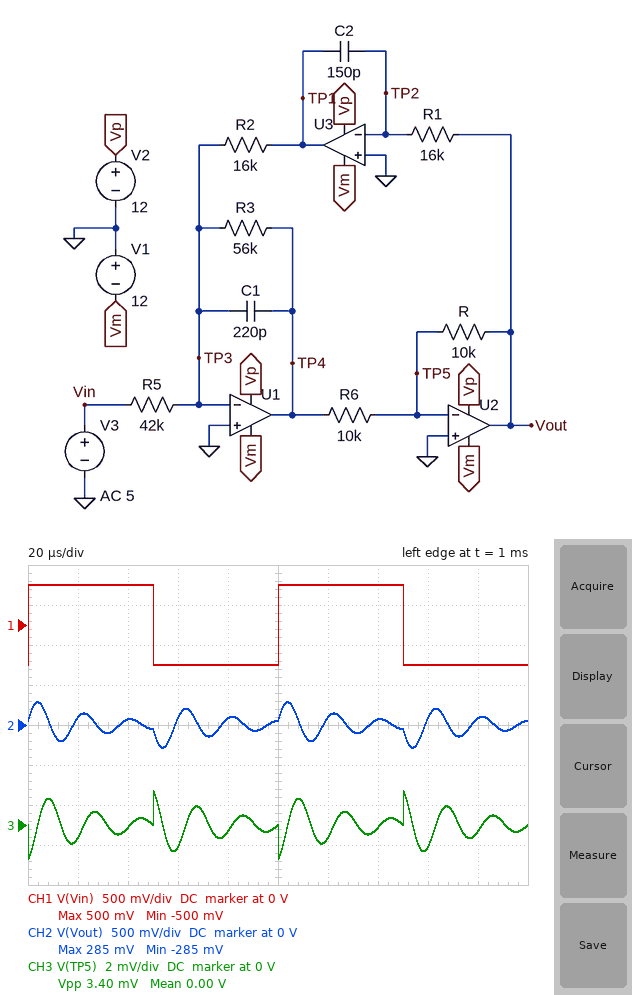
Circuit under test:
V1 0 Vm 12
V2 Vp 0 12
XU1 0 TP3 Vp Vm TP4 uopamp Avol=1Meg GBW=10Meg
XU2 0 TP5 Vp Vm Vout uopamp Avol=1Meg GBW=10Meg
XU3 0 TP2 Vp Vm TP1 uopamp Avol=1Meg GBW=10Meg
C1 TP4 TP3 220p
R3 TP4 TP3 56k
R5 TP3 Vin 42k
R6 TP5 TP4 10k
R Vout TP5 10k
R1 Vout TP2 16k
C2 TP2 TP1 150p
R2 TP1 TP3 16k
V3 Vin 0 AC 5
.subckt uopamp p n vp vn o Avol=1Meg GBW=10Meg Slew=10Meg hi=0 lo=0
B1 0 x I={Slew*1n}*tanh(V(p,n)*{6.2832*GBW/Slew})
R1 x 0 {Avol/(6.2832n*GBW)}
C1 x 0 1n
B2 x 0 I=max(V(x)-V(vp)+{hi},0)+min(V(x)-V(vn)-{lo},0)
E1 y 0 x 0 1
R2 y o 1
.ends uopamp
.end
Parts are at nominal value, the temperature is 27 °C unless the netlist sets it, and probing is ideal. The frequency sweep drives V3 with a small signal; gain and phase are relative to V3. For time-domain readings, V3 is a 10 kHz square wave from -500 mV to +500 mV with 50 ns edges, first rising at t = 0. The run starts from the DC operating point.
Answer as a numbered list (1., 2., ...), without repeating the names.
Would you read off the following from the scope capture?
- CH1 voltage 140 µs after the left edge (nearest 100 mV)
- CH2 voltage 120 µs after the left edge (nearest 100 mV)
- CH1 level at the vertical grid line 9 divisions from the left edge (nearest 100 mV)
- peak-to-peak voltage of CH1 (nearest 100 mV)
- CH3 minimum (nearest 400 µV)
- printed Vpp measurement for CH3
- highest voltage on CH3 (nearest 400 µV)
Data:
1. 500 mV
2. 100 mV
3. -500 mV
4. 1.0 V
5. -1.6 mV
6. 3.40 mV
7. 1.6 mV
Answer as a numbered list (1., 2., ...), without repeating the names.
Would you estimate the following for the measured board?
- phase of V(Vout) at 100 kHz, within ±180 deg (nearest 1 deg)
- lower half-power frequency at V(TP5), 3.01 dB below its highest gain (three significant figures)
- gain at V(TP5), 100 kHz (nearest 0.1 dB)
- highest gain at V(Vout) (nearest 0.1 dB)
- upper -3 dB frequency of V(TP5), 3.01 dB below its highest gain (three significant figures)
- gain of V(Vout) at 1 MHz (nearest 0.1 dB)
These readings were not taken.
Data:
1. -82 deg
2. 49.9 kHz
3. -52.4 dB
4. 3.3 dB
5. 62.2 kHz
6. -35.5 dB
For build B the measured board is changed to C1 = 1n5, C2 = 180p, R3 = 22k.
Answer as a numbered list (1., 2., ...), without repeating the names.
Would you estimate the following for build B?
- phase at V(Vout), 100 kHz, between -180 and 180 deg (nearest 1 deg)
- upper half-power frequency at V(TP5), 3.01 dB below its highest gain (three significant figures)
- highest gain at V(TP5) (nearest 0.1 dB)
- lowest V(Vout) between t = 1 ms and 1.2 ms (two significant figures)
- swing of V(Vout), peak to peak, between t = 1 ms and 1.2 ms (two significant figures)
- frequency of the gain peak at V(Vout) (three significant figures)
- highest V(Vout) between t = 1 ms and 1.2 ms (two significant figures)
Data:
1. -89 deg
2. 22.4 kHz
3. -59.7 dB
4. -77 mV
5. 150 mV
6. 19.1 kHz
7. 77 mV
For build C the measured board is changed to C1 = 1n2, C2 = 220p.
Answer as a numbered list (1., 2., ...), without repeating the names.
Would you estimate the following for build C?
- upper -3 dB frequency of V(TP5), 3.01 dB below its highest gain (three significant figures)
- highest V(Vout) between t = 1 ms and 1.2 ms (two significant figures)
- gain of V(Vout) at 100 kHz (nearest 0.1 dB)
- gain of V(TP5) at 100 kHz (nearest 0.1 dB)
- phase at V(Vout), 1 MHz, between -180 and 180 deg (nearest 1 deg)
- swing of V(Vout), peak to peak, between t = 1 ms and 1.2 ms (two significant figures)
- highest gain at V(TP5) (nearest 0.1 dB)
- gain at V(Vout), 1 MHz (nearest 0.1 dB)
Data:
1. 20.6 kHz
2. 89 mV
3. -29.7 dB
4. -69.7 dB
5. -107 deg
6. 180 mV
7. -51.2 dB
8. -50.2 dB
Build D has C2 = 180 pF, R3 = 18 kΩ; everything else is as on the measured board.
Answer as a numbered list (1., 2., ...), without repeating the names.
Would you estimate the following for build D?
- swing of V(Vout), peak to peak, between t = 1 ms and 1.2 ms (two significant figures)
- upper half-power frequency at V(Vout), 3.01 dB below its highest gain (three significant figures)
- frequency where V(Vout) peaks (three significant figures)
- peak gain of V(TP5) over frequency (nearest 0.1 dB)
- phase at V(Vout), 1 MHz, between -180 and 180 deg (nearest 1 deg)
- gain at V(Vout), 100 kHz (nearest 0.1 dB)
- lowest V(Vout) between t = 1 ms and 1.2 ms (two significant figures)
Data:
1. 420 mV
2. 72.8 kHz
3. 49.7 kHz
4. -52.5 dB
5. -105 deg
6. -13.9 dB
7. -210 mV
